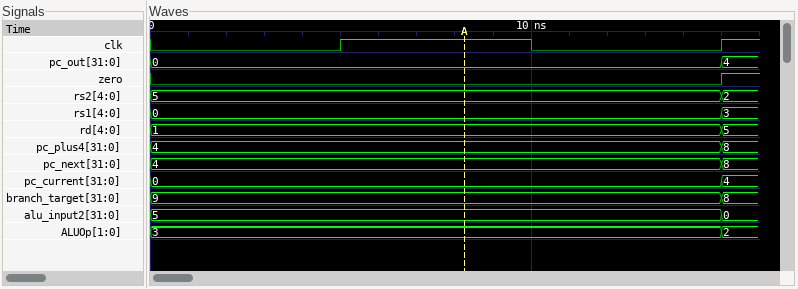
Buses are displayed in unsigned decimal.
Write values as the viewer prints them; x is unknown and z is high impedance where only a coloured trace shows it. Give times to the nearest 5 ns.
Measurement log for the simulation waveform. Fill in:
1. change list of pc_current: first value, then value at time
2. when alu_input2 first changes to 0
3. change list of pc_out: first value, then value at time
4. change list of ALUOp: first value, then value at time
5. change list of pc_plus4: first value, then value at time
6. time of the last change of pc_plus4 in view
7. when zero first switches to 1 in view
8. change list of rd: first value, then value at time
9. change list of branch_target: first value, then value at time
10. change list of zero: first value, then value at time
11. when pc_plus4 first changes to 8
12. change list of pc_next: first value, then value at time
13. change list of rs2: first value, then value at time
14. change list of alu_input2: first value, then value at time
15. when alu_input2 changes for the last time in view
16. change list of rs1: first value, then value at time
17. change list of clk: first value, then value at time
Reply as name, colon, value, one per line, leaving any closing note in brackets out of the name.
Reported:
change list of pc_current: first value, then value at time: 0, 4 at 15 ns
when alu_input2 first changes to 0: 15 ns
change list of pc_out: first value, then value at time: 0, 4 at 15 ns
change list of ALUOp: first value, then value at time: 3, 2 at 15 ns
change list of pc_plus4: first value, then value at time: 4, 8 at 15 ns
time of the last change of pc_plus4 in view: 15 ns
when zero first switches to 1 in view: 15 ns
change list of rd: first value, then value at time: 1, 5 at 15 ns
change list of branch_target: first value, then value at time: 9, 8 at 15 ns
change list of zero: first value, then value at time: 0, 1 at 15 ns
when pc_plus4 first changes to 8: 15 ns
change list of pc_next: first value, then value at time: 4, 8 at 15 ns
change list of rs2: first value, then value at time: 5, 2 at 15 ns
change list of alu_input2: first value, then value at time: 5, 0 at 15 ns
when alu_input2 changes for the last time in view: 15 ns
change list of rs1: first value, then value at time: 0, 3 at 15 ns
change list of clk: first value, then value at time: 0, 1 at 5 ns, 0 at 10 ns, 1 at 15 ns
